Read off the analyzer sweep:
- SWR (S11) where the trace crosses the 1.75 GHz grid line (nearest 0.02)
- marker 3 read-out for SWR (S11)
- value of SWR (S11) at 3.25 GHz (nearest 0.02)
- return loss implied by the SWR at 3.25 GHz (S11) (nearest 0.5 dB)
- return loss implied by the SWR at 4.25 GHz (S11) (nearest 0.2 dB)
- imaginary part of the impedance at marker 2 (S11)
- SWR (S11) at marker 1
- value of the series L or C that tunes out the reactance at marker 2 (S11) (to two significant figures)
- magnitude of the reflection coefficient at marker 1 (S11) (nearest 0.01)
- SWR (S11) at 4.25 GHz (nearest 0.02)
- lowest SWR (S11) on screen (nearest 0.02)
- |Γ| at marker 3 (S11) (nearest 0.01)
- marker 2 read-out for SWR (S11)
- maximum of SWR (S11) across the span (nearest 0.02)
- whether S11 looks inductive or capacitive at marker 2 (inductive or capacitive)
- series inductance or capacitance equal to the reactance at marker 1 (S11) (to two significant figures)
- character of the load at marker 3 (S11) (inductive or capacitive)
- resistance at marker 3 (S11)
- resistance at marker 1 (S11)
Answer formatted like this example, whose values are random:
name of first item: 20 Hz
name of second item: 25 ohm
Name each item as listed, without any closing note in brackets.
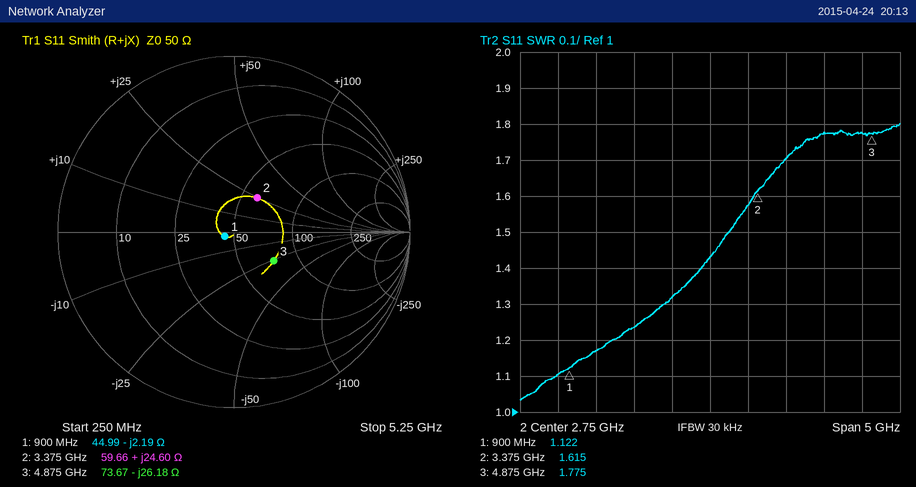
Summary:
SWR (S11) where the trace crosses the 1.75 GHz grid line: 1.24
marker 3 read-out for SWR: 1.775
value of SWR (S11) at 3.25 GHz: 1.58
return loss implied by the SWR at 3.25 GHz (S11): 13.0 dB
return loss implied by the SWR at 4.25 GHz (S11): 11.0 dB
imaginary part of the impedance at marker 2: +24.60 Ω
SWR (S11) at marker 1: 1.122
value of the series L or C that tunes out the reactance at marker 2 (S11): 1.9 pF
magnitude of the reflection coefficient at marker 1 (S11): 0.06
SWR (S11) at 4.25 GHz: 1.78
lowest SWR (S11) on screen: 1.04
|Γ| at marker 3 (S11): 0.28
marker 2 read-out for SWR: 1.615
maximum of SWR (S11) across the span: 1.80
whether S11 looks inductive or capacitive at marker 2: inductive
series inductance or capacitance equal to the reactance at marker 1 (S11): 81 pF
character of the load at marker 3 (S11): capacitive
resistance at marker 3: 73.67 Ω
resistance at marker 1: 44.99 Ω
